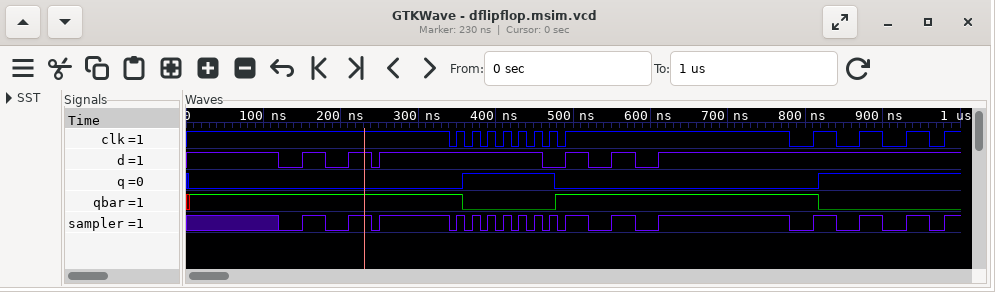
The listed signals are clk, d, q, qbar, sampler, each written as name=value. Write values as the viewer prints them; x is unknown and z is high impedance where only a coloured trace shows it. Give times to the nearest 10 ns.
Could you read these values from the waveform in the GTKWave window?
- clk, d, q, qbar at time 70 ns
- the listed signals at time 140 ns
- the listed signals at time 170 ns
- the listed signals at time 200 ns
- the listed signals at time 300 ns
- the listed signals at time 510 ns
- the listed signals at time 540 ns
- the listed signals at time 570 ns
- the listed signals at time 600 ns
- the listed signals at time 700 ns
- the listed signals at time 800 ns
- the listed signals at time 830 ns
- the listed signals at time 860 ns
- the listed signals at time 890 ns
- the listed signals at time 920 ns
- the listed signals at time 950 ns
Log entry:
clk=1, d=1, q=0, qbar=1
clk=1, d=0, q=0, qbar=1, sampler=0
clk=1, d=1, q=0, qbar=1, sampler=1
clk=1, d=0, q=0, qbar=1, sampler=0
clk=1, d=1, q=0, qbar=1, sampler=1
clk=1, d=1, q=0, qbar=1, sampler=1
clk=1, d=0, q=0, qbar=1, sampler=0
clk=1, d=1, q=0, qbar=1, sampler=1
clk=1, d=0, q=0, qbar=1, sampler=0
clk=1, d=1, q=0, qbar=1, sampler=1
clk=0, d=1, q=0, qbar=1, sampler=0
clk=1, d=1, q=1, qbar=0, sampler=1
clk=0, d=1, q=1, qbar=0, sampler=0
clk=1, d=1, q=1, qbar=0, sampler=1
clk=0, d=1, q=1, qbar=0, sampler=0
clk=1, d=1, q=1, qbar=0, sampler=1
